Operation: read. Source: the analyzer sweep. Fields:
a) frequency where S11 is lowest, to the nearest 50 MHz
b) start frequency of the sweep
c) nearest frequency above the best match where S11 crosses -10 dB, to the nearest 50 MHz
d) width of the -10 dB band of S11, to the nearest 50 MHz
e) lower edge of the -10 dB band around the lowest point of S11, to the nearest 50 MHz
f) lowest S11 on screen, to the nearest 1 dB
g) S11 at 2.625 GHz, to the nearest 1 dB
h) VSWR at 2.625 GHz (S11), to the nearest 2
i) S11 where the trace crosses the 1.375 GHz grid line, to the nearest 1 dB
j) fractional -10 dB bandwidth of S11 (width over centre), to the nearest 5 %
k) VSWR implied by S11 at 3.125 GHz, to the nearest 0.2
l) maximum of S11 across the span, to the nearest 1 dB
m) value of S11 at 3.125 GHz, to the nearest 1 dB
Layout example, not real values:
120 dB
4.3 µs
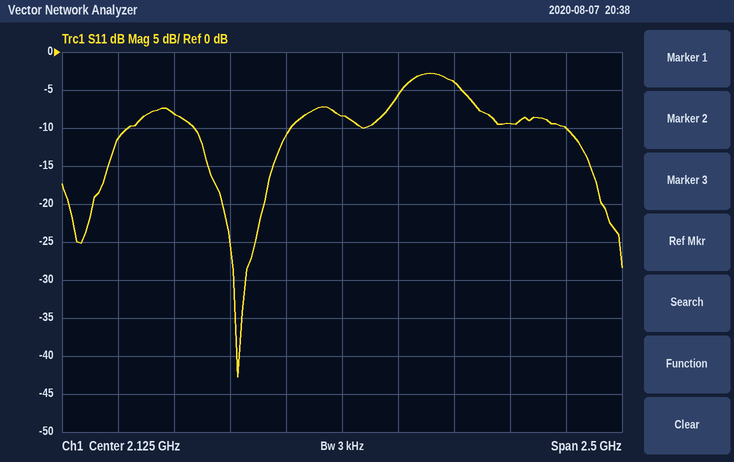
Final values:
1.65 GHz
875 MHz
1.90 GHz
450 MHz
1.45 GHz
-43 dB
-4 dB
4
-8 dB
25 %
2.0
-3 dB
-10 dB
